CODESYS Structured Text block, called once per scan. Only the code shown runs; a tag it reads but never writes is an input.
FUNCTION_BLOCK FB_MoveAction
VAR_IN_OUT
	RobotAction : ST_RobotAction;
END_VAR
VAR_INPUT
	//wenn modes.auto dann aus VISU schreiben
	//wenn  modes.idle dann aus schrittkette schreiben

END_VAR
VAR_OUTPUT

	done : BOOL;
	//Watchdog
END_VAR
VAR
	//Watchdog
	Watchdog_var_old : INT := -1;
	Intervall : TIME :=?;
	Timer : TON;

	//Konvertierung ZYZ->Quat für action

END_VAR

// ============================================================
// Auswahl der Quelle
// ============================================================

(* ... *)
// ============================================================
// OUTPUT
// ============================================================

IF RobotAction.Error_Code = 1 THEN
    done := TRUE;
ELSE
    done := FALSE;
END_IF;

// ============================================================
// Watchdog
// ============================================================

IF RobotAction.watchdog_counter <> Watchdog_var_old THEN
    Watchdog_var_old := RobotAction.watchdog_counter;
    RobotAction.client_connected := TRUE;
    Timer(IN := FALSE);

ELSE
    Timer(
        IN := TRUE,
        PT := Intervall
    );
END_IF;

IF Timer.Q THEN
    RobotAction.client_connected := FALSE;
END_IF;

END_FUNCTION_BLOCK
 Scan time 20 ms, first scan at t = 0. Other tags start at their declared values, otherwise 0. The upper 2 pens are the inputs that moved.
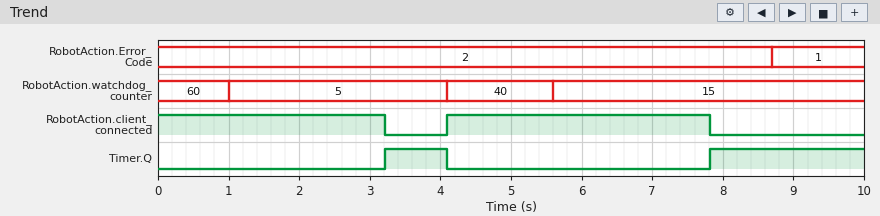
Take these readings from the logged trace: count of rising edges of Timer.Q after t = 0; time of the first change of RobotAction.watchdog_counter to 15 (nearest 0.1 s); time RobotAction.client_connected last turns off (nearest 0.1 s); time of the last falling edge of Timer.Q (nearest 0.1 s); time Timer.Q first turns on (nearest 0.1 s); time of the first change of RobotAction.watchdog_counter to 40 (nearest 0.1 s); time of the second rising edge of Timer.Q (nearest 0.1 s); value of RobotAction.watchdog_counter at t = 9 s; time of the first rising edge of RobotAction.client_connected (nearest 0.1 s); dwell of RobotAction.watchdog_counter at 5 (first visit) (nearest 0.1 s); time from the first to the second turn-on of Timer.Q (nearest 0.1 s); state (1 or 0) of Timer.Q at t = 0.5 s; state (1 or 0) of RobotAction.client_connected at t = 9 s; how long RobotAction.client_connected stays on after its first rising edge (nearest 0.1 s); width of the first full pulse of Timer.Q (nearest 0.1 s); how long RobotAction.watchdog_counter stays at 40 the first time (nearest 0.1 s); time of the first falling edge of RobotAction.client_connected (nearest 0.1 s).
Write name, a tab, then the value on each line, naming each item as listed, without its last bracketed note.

count of rising edges of Timer.Q after t = 0	2
time of the first change of RobotAction.watchdog_counter to 15	5.6 s
time RobotAction.client_connected last turns off	7.8 s
time of the last falling edge of Timer.Q	4.1 s
time Timer.Q first turns on	3.2 s
time of the first change of RobotAction.watchdog_counter to 40	4.1 s
time of the second rising edge of Timer.Q	7.8 s
value of RobotAction.watchdog_counter at t = 9 s	15
time of the first rising edge of RobotAction.client_connected	4.1 s
dwell of RobotAction.watchdog_counter at 5 (first visit)	3.1 s
time from the first to the second turn-on of Timer.Q	4.6 s
state (1 or 0) of Timer.Q at t = 0.5 s	0
state (1 or 0) of RobotAction.client_connected at t = 9 s	0
how long RobotAction.client_connected stays on after its first rising edge	3.7 s
width of the first full pulse of Timer.Q	0.9 s
how long RobotAction.watchdog_counter stays at 40 the first time	1.5 s
time of the first falling edge of RobotAction.client_connected	3.2 s
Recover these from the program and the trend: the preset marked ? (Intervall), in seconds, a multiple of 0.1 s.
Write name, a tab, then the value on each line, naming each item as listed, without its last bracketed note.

the preset marked ? (Intervall), in seconds, a multiple of 0.1 s	2.2 s
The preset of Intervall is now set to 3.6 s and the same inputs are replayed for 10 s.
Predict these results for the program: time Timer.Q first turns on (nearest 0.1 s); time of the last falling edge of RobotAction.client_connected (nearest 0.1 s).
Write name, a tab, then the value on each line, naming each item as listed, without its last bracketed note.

time Timer.Q first turns on	9.2 s
time of the last falling edge of RobotAction.client_connected	9.2 s
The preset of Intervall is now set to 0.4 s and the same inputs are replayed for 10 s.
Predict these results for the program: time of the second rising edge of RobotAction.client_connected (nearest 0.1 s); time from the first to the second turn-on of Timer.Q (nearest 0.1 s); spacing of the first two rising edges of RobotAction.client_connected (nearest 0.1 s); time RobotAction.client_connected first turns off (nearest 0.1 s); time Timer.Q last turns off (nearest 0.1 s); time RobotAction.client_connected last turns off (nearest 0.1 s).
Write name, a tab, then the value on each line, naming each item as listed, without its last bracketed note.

time of the second rising edge of RobotAction.client_connected	4.1 s
time from the first to the second turn-on of Timer.Q	1.0 s
spacing of the first two rising edges of RobotAction.client_connected	3.1 s
time RobotAction.client_connected first turns off	0.4 s
time Timer.Q last turns off	5.6 s
time RobotAction.client_connected last turns off	6.0 s
